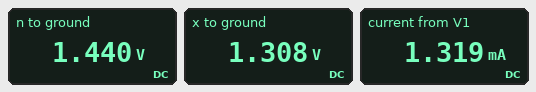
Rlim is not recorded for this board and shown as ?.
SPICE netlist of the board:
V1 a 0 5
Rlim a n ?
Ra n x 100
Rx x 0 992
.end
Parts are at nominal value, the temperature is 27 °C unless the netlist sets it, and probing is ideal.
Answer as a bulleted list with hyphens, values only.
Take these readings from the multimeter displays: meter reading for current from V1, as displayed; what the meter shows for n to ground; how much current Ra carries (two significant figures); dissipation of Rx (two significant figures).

- 1.319 mA
- 1.440 V
- 1.3 mA
- 1.7 mW
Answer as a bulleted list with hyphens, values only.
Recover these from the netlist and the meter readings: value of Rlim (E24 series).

- 2.7 kΩ
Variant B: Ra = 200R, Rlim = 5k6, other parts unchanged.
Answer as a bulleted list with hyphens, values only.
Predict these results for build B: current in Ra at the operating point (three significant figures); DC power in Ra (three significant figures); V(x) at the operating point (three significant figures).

- 736 µA
- 108 µW
- 730 mV
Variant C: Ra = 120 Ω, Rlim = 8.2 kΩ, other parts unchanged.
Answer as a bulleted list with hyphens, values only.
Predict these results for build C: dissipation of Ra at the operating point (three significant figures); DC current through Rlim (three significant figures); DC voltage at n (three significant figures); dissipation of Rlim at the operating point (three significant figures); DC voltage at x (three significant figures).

- 34.6 µW
- 537 µA
- 597 mV
- 2.36 mW
- 533 mV
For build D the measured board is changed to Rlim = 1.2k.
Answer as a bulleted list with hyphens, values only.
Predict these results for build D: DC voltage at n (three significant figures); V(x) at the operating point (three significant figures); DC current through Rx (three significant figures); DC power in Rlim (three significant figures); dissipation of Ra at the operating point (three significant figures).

- 2.38 V
- 2.16 V
- 2.18 mA
- 5.71 mW
- 476 µW
